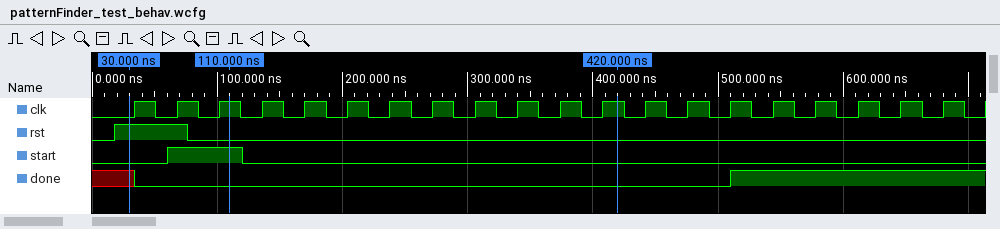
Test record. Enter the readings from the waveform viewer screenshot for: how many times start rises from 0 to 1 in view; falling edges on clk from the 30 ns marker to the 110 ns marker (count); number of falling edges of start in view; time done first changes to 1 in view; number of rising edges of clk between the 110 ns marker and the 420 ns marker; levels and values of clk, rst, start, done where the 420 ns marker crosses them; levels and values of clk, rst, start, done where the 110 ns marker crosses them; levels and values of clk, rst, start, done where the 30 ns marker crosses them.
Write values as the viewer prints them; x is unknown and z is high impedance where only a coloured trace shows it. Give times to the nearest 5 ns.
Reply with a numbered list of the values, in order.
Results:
1. 1
2. 2
3. 1
4. 510 ns
5. 9
6. clk=1, rst=0, start=0, done=0
7. clk=1, rst=0, start=1, done=0
8. clk=0, rst=1, start=0, done=x
